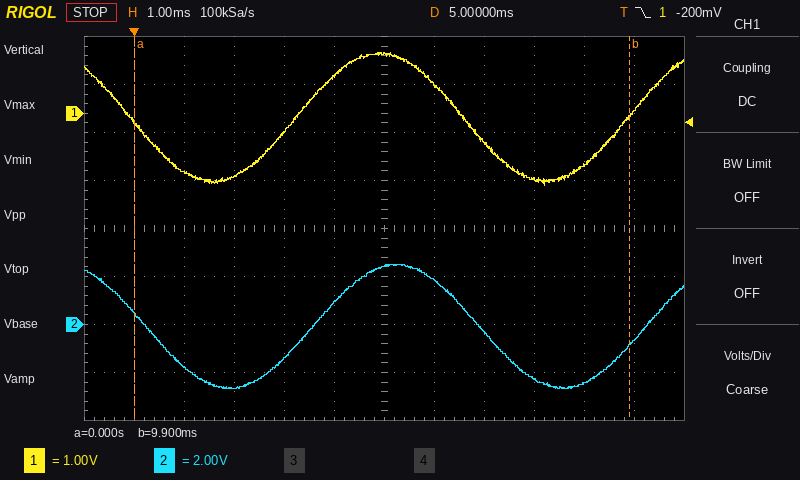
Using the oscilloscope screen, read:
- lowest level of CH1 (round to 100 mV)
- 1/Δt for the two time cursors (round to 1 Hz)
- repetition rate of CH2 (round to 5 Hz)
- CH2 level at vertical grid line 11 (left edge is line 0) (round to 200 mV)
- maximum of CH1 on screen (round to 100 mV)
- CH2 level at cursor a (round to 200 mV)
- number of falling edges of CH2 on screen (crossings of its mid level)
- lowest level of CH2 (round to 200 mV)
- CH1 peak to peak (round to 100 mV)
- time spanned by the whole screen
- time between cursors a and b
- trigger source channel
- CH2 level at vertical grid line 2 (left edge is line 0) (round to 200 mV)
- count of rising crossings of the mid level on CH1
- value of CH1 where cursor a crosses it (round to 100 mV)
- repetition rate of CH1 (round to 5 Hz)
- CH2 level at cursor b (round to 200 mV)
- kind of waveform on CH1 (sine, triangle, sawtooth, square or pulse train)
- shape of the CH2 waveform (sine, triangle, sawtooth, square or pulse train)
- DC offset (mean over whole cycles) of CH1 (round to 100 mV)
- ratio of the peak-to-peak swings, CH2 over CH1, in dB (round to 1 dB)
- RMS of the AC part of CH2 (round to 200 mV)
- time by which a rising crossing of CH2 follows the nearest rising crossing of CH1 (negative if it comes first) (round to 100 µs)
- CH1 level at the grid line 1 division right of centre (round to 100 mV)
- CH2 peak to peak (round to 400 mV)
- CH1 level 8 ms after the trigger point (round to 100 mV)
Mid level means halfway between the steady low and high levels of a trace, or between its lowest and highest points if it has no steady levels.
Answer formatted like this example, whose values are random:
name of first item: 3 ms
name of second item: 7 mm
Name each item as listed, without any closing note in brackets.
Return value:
lowest level of CH1: -1.5 V
1/Δt for the two time cursors: 101 Hz
repetition rate of CH2: 150 Hz
CH2 level at vertical grid line 11 (left edge is line 0): -600 mV
maximum of CH1 on screen: 1.3 V
CH2 level at cursor a: 400 mV
number of falling edges of CH2 on screen: 2
lowest level of CH2: -2.6 V
CH1 peak to peak: 2.8 V
time spanned by the whole screen: 12 ms
time between cursors a and b: 9.9 ms
trigger source channel: CH1
CH2 level at vertical grid line 2 (left edge is line 0): -1.8 V
count of rising crossings of the mid level on CH1: 2
value of CH1 where cursor a crosses it: -200 mV
repetition rate of CH1: 150 Hz
CH2 level at cursor b: -800 mV
kind of waveform on CH1: sine
shape of the CH2 waveform: sine
DC offset (mean over whole cycles) of CH1: -100 mV
ratio of the peak-to-peak swings, CH2 over CH1, in dB: 5 dB
RMS of the AC part of CH2: 1.8 V
time by which a rising crossing of CH2 follows the nearest rising crossing of CH1 (negative if it comes first): +400 µs
CH1 level at the grid line 1 division right of centre: 600 mV
CH2 peak to peak: 5.2 V
CH1 level 8 ms after the trigger point: -1.4 V
